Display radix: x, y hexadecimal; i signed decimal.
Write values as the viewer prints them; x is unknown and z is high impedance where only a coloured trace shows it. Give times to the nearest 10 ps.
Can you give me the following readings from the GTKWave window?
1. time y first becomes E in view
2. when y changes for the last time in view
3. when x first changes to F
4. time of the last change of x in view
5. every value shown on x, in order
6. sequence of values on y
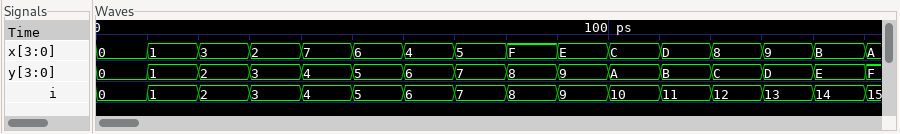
140 ps
150 ps
80 ps
150 ps
0, 1, 3, 2, 7, 6, 4, 5, F, E, C, D, 8, 9, B, A
0, 1, 2, 3, 4, 5, 6, 7, 8, 9, A, B, C, D, E, F
